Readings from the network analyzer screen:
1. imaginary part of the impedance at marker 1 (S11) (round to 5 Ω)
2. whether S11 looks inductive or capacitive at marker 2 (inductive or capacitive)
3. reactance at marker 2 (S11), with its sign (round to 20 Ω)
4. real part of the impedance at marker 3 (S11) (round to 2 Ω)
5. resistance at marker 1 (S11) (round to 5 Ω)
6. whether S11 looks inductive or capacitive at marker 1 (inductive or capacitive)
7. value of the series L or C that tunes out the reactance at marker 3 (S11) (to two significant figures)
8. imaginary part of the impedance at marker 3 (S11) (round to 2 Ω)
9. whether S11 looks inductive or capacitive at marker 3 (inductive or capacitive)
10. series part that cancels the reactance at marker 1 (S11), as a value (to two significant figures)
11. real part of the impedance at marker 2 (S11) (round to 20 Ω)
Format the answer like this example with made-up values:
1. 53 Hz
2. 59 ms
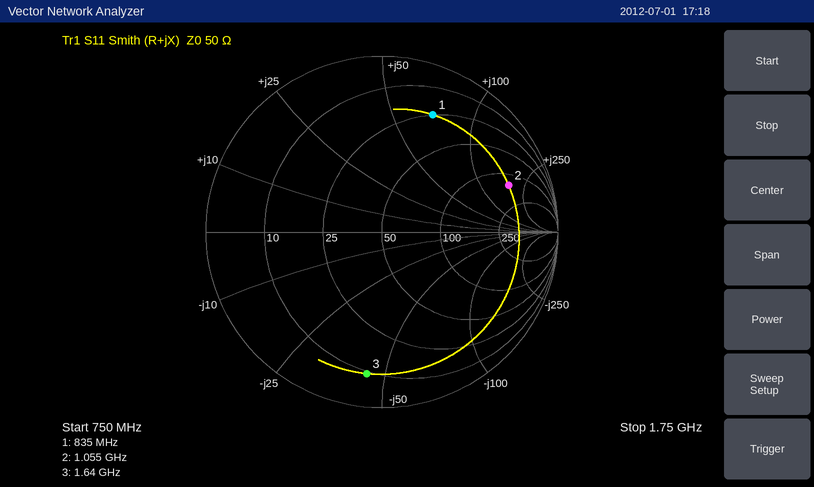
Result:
1. +70 Ω
2. inductive
3. +180 Ω
4. 10 Ω
5. 25 Ω
6. inductive
7. 4.3 nH
8. -44 Ω
9. capacitive
10. 2.7 pF
11. 140 Ω
